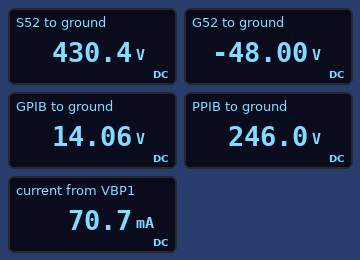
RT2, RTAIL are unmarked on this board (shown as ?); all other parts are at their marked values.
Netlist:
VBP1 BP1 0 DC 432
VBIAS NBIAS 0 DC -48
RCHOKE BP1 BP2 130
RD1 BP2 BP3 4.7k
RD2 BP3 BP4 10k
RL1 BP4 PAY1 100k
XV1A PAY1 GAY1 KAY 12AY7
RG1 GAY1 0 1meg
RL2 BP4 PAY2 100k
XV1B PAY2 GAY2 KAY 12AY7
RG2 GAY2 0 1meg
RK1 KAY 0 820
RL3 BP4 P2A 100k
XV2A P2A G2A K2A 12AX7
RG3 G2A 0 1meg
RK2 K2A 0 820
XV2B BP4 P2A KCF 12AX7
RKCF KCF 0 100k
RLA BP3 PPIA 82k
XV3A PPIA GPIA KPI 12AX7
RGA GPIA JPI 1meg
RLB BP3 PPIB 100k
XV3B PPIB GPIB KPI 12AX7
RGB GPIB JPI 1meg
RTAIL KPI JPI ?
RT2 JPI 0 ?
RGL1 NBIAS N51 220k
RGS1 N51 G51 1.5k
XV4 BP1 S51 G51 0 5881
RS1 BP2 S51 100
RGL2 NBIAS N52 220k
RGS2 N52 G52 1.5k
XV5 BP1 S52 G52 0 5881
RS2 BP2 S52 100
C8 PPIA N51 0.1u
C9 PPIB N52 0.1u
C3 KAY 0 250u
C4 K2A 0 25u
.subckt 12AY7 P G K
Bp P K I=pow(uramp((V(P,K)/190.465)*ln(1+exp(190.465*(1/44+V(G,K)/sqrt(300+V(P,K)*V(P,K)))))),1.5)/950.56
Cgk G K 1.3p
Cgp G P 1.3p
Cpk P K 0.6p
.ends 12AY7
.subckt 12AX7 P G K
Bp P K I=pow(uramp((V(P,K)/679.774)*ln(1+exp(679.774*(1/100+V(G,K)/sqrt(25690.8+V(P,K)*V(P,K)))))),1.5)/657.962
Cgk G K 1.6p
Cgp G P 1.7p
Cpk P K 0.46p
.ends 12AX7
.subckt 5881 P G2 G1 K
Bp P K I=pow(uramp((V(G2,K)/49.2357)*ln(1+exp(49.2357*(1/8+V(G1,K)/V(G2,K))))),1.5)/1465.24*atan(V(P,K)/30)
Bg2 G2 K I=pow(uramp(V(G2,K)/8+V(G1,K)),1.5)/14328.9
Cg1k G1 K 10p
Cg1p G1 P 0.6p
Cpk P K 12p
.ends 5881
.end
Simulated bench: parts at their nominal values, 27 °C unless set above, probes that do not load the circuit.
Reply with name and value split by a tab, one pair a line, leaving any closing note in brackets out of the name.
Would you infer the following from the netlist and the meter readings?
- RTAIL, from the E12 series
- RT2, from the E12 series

RTAIL, from the E12 series	560 Ω
RT2, from the E12 series	4.7 kΩ
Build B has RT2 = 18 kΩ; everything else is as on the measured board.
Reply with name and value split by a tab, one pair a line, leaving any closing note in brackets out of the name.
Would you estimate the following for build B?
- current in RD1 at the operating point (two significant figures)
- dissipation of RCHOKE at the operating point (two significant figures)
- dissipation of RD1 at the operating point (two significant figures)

current in RD1 at the operating point	9.1 mA
dissipation of RCHOKE at the operating point	16 mW
dissipation of RD1 at the operating point	390 mW
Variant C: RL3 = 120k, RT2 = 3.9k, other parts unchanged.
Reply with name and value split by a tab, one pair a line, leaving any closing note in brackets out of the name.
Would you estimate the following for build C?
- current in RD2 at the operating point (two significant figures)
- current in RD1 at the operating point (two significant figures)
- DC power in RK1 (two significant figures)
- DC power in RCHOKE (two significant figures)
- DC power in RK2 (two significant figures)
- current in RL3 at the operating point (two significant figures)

current in RD2 at the operating point	6.2 mA
current in RD1 at the operating point	9.2 mA
DC power in RK1	8.3 mW
DC power in RCHOKE	16 mW
DC power in RK2	1.4 mW
current in RL3 at the operating point	1.3 mA
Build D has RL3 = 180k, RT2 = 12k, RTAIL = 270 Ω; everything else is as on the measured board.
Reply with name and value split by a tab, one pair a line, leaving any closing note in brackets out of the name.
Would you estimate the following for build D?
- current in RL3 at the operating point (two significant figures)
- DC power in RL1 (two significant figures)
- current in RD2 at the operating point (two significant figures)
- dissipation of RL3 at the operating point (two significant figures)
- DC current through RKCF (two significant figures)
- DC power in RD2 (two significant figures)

current in RL3 at the operating point	1.1 mA
DC power in RL1	260 mW
current in RD2 at the operating point	5.7 mA
dissipation of RL3 at the operating point	210 mW
DC current through RKCF	1.4 mA
DC power in RD2	320 mW
